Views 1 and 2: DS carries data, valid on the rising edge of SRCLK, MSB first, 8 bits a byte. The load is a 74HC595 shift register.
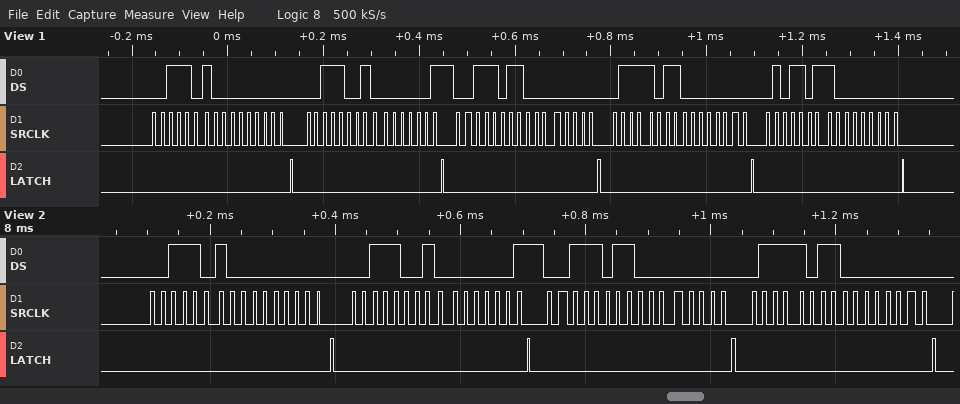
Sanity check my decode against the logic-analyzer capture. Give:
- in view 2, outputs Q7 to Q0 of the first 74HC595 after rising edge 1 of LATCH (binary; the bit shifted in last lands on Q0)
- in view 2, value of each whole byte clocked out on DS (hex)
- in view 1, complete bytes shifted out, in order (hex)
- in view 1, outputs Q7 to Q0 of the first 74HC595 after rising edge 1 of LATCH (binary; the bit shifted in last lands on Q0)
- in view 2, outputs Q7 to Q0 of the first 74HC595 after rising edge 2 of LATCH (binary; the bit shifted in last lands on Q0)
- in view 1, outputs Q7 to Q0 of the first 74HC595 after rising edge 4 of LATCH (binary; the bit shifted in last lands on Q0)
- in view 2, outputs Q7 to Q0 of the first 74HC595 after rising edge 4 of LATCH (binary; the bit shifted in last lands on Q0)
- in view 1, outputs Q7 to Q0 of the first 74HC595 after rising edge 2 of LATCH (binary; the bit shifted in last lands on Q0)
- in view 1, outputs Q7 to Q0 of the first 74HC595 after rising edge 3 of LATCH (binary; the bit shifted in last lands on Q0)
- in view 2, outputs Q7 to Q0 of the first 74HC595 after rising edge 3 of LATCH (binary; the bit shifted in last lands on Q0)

00000000
3A 00 39 01 3B 00 7B 00
3A 00 39 01 3B 00 7B 00 5B 00
00000000
00000001
00000000
00000000
00000001
00000000
00000000
